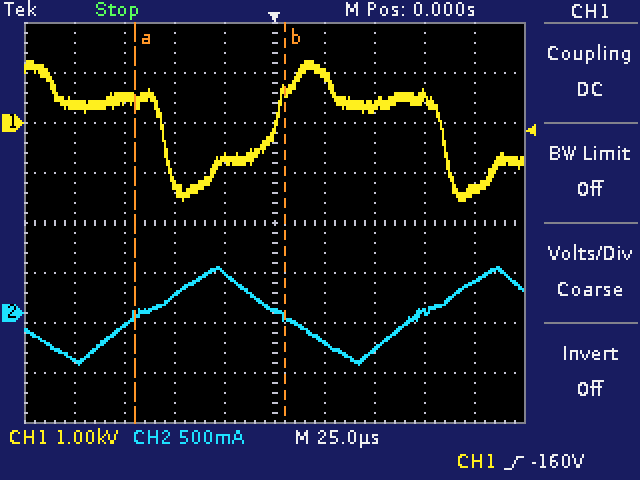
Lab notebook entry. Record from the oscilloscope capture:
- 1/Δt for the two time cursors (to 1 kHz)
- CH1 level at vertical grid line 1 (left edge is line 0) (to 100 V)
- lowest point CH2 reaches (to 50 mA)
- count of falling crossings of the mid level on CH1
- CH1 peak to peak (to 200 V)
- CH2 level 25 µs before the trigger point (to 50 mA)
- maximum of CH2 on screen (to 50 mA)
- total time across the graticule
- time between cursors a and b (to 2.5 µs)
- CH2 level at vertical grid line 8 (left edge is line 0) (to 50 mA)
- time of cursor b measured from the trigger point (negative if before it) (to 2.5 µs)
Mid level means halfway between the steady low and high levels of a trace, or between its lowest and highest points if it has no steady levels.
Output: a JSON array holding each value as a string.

["13 kHz", "400 V", "-500 mA", "2", "2.8 kV", "400 mA", "450 mA", "250 µs", "75.0 µs", "0 mA", "+5.0 µs"]
